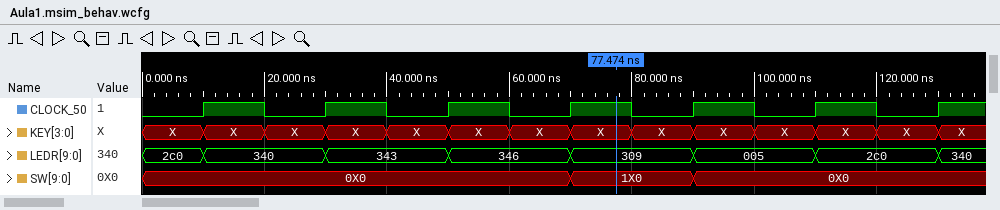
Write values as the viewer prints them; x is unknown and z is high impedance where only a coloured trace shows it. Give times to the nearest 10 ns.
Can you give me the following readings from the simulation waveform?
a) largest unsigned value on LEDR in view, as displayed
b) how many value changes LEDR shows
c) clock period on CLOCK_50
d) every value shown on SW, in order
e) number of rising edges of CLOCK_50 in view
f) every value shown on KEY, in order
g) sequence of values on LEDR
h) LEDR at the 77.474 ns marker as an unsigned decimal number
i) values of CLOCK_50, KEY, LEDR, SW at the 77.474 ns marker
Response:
346
7
20 ns
0X0, 1X0, 0X0
7
X, X, X, X, X, X, X, X, X, X, X, X, X, X
2c0, 340, 343, 346, 309, 005, 2c0, 340
777
CLOCK_50=1, KEY=X, LEDR=309, SW=1X0
